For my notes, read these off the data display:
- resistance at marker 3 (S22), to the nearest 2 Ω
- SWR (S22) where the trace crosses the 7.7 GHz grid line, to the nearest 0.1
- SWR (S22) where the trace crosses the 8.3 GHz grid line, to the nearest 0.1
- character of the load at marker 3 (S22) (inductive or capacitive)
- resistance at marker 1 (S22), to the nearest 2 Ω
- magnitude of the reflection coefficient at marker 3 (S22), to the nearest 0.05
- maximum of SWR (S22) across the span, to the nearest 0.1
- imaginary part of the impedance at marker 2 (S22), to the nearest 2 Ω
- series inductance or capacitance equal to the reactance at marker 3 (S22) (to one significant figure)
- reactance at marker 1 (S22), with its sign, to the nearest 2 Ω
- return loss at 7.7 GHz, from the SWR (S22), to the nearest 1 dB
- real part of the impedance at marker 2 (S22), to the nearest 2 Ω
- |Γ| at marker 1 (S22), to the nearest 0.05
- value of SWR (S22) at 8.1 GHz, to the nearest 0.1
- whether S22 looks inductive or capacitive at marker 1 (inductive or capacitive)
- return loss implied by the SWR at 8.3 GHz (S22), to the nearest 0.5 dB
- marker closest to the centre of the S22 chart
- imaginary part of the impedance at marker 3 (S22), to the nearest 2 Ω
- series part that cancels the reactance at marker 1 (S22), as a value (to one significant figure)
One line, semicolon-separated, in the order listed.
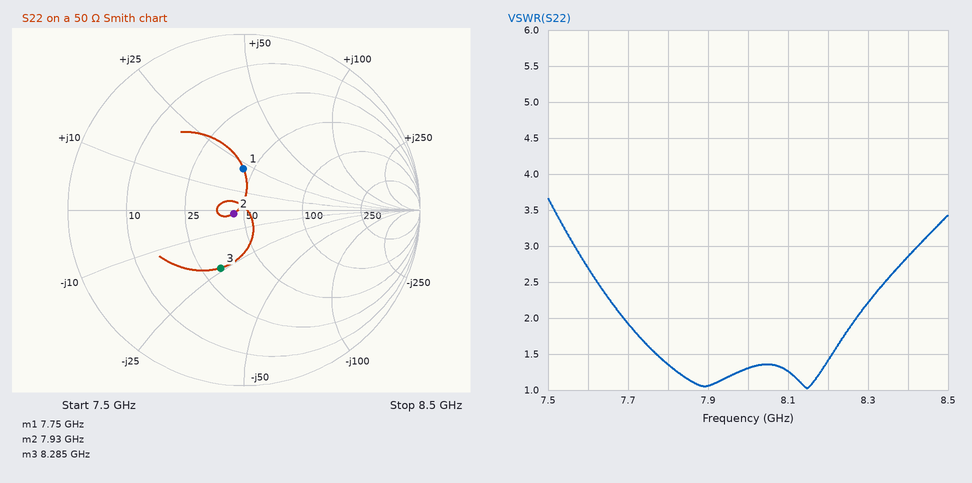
32 Ω; 1.9; 2.2; capacitive; 44 Ω; 0.35; 3.7; -2 Ω; 800 fF; +22 Ω; 10 dB; 44 Ω; 0.25; 1.3; inductive; 8.5 dB; marker 2; -24 Ω; 900 fF
